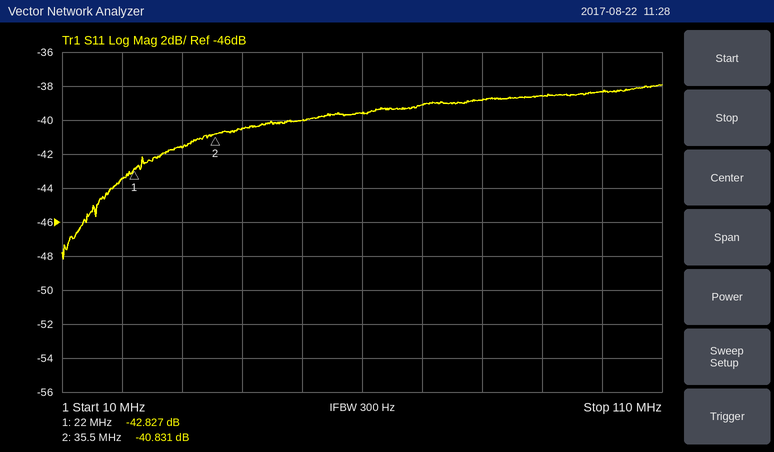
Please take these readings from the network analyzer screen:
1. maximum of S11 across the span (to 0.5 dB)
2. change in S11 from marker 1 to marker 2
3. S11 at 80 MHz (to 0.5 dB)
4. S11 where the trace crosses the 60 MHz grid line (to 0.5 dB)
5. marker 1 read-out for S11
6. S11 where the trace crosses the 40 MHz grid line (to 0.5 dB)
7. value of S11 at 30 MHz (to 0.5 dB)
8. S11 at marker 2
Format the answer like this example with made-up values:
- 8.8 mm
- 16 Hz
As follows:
- -38.0 dB
- 1.996 dB
- -39.0 dB
- -39.5 dB
- -42.827 dB
- -40.5 dB
- -41.5 dB
- -40.831 dB
